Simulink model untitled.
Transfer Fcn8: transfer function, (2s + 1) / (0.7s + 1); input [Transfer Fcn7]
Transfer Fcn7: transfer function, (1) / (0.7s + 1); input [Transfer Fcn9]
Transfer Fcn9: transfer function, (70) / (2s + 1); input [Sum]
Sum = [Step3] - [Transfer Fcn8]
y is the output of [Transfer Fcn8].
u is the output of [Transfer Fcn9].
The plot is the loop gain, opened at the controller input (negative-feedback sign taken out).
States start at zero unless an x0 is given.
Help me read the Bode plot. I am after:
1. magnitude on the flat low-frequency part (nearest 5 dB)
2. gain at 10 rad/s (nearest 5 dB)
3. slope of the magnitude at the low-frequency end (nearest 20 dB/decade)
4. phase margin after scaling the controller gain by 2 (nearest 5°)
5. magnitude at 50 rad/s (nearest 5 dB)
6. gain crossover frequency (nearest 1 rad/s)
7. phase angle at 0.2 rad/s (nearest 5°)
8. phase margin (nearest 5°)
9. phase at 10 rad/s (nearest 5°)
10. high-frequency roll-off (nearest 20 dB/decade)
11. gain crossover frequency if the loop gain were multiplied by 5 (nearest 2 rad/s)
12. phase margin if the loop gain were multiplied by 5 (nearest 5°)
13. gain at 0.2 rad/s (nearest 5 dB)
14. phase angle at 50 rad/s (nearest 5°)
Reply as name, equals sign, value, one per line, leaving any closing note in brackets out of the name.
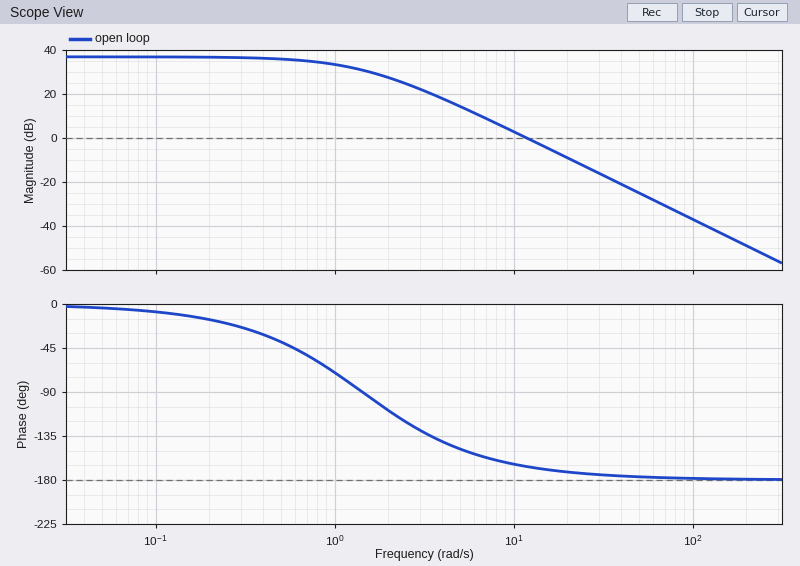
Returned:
magnitude on the flat low-frequency part = 35 dB
gain at 10 rad/s = 5 dB
slope of the magnitude at the low-frequency end = 0 dB/decade
phase margin after scaling the controller gain by 2 = 10°
magnitude at 50 rad/s = -25 dB
gain crossover frequency = 12 rad/s
phase angle at 0.2 rad/s = -15°
phase margin = 15°
phase at 10 rad/s = -165°
high-frequency roll-off = -40 dB/decade
gain crossover frequency if the loop gain were multiplied by 5 = 26 rad/s
phase margin if the loop gain were multiplied by 5 = 5°
gain at 0.2 rad/s = 35 dB
phase angle at 50 rad/s = -175°
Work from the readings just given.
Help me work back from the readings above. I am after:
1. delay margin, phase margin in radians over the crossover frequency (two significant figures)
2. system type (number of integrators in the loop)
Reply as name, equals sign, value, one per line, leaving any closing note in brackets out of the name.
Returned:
delay margin, phase margin in radians over the crossover frequency = 0.022 s
system type = 0
